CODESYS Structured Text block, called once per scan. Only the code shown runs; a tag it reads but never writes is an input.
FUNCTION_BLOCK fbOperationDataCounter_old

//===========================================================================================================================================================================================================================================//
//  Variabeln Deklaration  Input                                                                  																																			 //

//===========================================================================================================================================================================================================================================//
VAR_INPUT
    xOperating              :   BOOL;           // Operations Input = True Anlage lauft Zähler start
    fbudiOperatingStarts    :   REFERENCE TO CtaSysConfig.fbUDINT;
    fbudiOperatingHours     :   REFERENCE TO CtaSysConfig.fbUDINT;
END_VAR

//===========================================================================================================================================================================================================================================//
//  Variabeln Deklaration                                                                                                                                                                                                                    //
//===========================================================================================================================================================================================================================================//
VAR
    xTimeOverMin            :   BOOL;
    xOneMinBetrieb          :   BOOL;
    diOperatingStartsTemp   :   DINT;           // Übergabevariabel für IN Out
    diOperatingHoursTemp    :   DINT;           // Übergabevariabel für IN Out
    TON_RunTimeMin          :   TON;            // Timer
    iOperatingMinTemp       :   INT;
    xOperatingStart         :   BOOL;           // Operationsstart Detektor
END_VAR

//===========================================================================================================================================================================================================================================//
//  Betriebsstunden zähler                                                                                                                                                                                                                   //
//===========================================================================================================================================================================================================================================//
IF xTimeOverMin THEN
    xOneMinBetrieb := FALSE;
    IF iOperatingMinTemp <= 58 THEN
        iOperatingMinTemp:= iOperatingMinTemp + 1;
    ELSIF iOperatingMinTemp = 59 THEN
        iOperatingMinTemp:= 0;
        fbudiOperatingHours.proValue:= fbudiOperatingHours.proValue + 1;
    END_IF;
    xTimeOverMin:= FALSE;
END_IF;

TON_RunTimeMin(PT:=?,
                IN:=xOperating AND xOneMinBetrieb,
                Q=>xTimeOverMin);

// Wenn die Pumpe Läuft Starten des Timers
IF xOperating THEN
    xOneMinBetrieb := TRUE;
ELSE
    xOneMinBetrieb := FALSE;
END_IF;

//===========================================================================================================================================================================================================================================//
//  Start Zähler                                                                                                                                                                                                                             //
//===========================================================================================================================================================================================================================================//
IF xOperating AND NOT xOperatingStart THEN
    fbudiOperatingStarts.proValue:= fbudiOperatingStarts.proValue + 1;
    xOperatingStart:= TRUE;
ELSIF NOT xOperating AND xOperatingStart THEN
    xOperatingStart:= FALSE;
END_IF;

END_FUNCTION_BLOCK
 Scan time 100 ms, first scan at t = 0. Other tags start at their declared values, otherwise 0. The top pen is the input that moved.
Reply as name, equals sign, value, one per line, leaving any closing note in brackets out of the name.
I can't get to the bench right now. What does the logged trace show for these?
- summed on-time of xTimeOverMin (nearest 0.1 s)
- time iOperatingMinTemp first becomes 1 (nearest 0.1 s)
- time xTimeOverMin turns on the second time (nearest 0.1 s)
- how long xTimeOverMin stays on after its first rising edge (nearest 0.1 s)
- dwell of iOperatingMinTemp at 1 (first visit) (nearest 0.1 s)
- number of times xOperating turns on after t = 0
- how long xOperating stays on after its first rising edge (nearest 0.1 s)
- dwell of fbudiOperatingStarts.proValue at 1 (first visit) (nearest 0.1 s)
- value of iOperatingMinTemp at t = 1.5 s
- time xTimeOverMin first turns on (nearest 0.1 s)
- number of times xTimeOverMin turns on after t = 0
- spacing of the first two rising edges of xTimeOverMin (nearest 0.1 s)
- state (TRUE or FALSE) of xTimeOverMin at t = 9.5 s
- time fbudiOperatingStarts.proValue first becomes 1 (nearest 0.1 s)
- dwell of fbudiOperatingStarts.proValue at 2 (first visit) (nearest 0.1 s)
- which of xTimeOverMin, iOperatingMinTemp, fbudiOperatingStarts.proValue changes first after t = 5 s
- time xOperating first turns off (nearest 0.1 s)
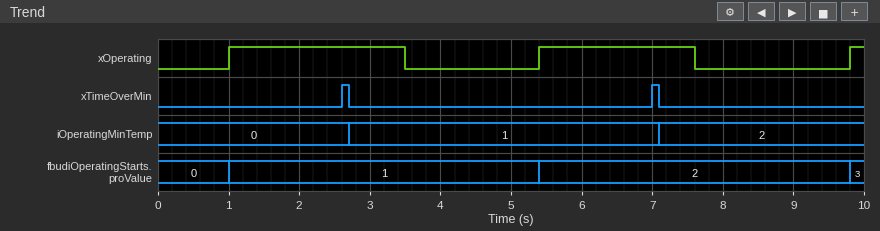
summed on-time of xTimeOverMin = 0.2 s
time iOperatingMinTemp first becomes 1 = 2.7 s
time xTimeOverMin turns on the second time = 7.0 s
how long xTimeOverMin stays on after its first rising edge = 0.1 s
dwell of iOperatingMinTemp at 1 (first visit) = 4.4 s
number of times xOperating turns on after t = 0 = 3
how long xOperating stays on after its first rising edge = 2.5 s
dwell of fbudiOperatingStarts.proValue at 1 (first visit) = 4.4 s
value of iOperatingMinTemp at t = 1.5 s = 0
time xTimeOverMin first turns on = 2.6 s
number of times xTimeOverMin turns on after t = 0 = 2
spacing of the first two rising edges of xTimeOverMin = 4.4 s
state (TRUE or FALSE) of xTimeOverMin at t = 9.5 s = FALSE
time fbudiOperatingStarts.proValue first becomes 1 = 1.0 s
dwell of fbudiOperatingStarts.proValue at 2 (first visit) = 4.4 s
which of xTimeOverMin, iOperatingMinTemp, fbudiOperatingStarts.proValue changes first after t = 5 s = fbudiOperatingStarts.proValue
time xOperating first turns off = 3.5 s
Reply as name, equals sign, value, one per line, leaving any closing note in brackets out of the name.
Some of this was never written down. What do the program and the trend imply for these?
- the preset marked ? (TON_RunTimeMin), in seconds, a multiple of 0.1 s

the preset marked ? (TON_RunTimeMin), in seconds, a multiple of 0.1 s = 1.5 s
